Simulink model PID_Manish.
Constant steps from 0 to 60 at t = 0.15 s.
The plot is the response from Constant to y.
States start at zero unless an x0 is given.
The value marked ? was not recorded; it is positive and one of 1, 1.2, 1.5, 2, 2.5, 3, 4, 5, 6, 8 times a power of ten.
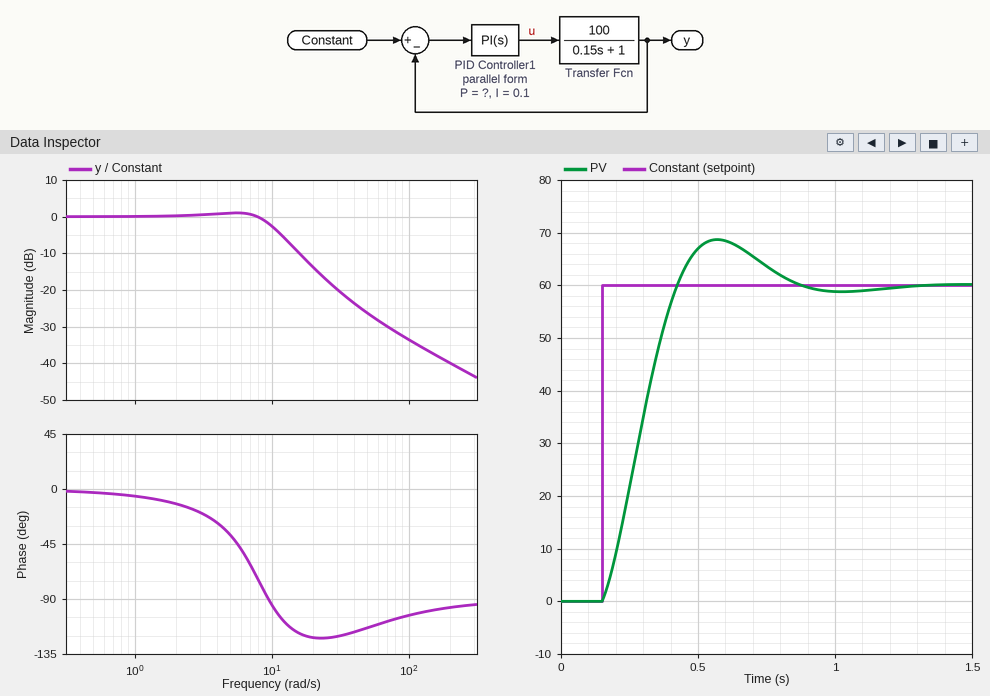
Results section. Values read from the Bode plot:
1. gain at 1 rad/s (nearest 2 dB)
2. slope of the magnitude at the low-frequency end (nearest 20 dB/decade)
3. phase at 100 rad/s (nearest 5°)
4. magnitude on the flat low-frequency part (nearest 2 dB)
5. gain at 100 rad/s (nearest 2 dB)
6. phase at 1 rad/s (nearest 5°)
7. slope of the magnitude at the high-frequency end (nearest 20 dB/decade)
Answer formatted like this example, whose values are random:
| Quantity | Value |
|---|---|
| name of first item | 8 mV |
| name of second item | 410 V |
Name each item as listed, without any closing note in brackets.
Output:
| Quantity | Value |
|---|---|
| gain at 1 rad/s | 0 dB |
| slope of the magnitude at the low-frequency end | 0 dB/decade |
| phase at 100 rad/s | -105° |
| magnitude on the flat low-frequency part | 0 dB |
| gain at 100 rad/s | -34 dB |
| phase at 1 rad/s | -5° |
| slope of the magnitude at the high-frequency end | -20 dB/decade |
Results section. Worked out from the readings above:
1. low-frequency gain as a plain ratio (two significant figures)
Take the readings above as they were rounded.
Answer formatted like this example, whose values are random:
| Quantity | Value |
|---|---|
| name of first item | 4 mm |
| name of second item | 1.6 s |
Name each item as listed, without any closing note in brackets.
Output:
| Quantity | Value |
|---|---|
| low-frequency gain as a plain ratio | 1.0 |
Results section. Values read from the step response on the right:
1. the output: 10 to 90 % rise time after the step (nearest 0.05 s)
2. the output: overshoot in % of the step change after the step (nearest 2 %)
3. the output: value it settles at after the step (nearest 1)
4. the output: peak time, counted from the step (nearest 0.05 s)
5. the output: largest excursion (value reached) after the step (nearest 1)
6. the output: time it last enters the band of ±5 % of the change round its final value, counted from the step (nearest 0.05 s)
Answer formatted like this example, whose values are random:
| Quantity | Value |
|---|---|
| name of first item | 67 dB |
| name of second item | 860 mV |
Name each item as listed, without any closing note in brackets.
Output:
| Quantity | Value |
|---|---|
| the output: 10 to 90 % rise time after the step | 0.20 s |
| the output: overshoot in % of the step change after the step | 14 % |
| the output: value it settles at after the step | 60 |
| the output: peak time, counted from the step | 0.40 s |
| the output: largest excursion (value reached) after the step | 69 |
| the output: time it last enters the band of ±5 % of the change round its final value, counted from the step | 0.60 s |
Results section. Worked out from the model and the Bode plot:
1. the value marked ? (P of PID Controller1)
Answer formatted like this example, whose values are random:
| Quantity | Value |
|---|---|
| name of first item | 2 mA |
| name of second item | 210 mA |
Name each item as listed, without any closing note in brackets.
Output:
| Quantity | Value |
|---|---|
| the value marked ? | 0.003 |
